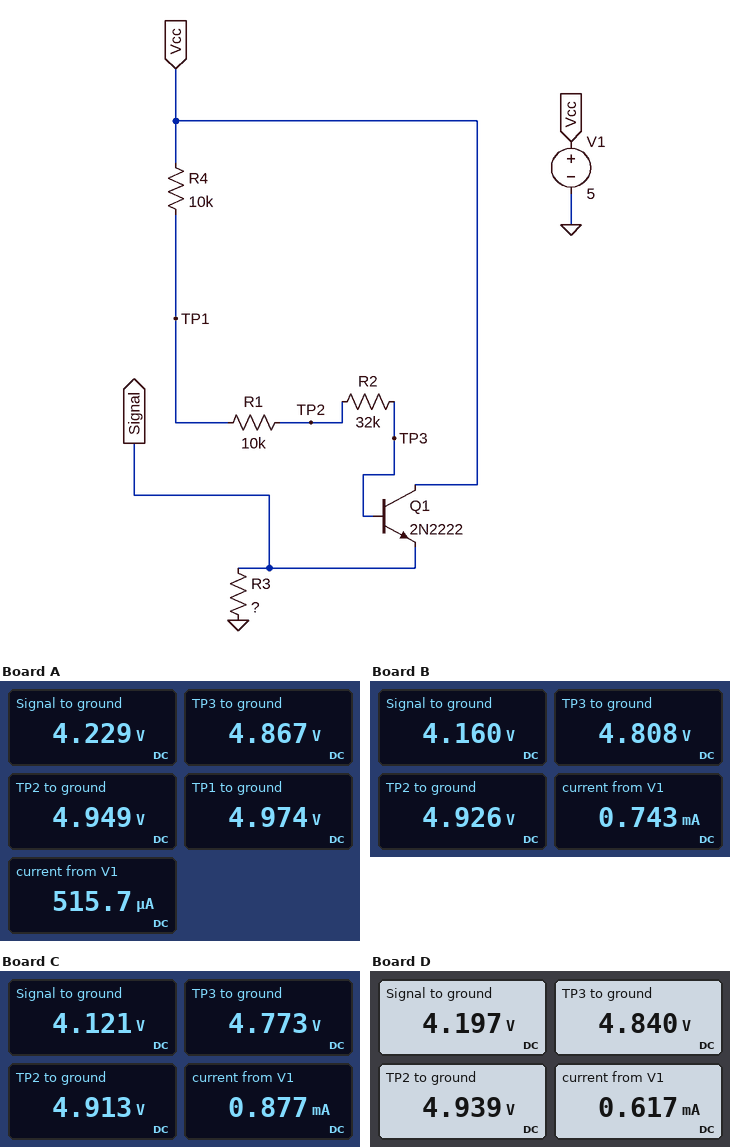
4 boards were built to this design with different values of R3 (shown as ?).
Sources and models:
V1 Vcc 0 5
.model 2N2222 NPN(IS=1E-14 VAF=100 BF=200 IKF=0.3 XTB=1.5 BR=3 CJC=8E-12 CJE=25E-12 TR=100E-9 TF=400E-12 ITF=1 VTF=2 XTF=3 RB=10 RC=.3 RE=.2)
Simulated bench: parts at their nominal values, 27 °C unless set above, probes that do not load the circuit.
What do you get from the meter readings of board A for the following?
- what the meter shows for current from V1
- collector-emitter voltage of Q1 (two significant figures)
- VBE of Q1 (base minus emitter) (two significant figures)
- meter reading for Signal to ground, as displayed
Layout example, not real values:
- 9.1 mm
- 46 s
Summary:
- 515.7 µA
- 770 mV
- 640 mV
- 4.229 V
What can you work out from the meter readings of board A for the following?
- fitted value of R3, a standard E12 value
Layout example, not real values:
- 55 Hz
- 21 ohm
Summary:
- 8.2 kΩ
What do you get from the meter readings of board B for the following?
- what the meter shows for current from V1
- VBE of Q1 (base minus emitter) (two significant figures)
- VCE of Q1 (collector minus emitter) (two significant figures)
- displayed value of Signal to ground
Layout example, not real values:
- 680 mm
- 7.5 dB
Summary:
- 0.743 mA
- 650 mV
- 840 mV
- 4.160 V
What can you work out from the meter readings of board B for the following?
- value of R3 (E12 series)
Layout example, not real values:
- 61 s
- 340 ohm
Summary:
- 5.6 kΩ
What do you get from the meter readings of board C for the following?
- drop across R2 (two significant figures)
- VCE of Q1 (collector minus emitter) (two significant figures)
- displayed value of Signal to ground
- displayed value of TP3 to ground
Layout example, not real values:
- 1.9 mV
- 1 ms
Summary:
- 140 mV
- 880 mV
- 4.121 V
- 4.773 V
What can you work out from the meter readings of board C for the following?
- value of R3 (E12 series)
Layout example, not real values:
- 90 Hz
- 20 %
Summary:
- 4.7 kΩ
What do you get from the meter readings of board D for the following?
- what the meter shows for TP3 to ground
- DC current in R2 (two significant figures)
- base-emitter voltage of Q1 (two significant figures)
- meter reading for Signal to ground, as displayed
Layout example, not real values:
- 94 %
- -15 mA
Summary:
- 4.840 V
- 3.1 µA
- 640 mV
- 4.197 V
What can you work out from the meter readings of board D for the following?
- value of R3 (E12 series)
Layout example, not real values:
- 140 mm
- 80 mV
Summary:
- 6.8 kΩ
